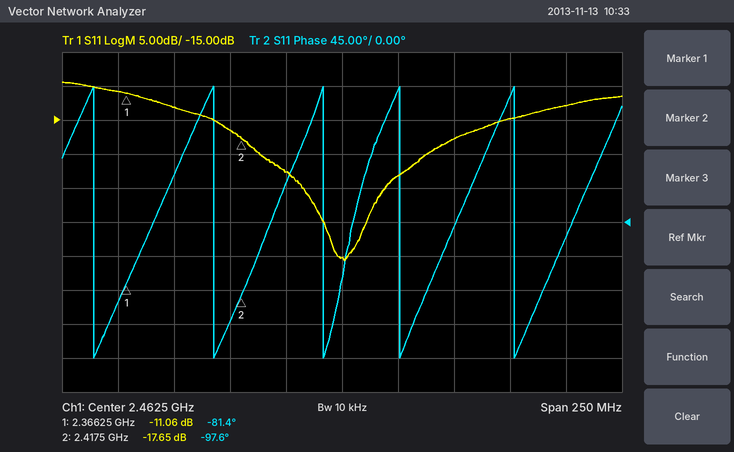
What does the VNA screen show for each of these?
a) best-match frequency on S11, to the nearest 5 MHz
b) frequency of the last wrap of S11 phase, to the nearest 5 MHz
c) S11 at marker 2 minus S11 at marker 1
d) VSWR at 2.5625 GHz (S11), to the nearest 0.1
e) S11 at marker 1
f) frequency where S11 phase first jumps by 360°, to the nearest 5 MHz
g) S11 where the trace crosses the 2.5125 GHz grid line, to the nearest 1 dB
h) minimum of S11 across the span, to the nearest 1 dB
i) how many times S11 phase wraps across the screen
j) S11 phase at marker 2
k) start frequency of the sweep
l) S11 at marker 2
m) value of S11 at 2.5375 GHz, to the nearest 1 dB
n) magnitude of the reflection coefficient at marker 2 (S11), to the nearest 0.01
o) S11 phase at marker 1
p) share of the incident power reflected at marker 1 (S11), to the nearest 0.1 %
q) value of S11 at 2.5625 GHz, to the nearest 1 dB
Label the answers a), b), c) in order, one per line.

a) 2.465 GHz
b) 2.540 GHz
c) -6.59 dB
d) 1.6
e) -11.06 dB
f) 2.350 GHz
g) -18 dB
h) -36 dB
i) 5
j) -97.6°
k) 2.3375 GHz
l) -17.65 dB
m) -15 dB
n) 0.13
o) -81.4°
p) 7.8 %
q) -13 dB
